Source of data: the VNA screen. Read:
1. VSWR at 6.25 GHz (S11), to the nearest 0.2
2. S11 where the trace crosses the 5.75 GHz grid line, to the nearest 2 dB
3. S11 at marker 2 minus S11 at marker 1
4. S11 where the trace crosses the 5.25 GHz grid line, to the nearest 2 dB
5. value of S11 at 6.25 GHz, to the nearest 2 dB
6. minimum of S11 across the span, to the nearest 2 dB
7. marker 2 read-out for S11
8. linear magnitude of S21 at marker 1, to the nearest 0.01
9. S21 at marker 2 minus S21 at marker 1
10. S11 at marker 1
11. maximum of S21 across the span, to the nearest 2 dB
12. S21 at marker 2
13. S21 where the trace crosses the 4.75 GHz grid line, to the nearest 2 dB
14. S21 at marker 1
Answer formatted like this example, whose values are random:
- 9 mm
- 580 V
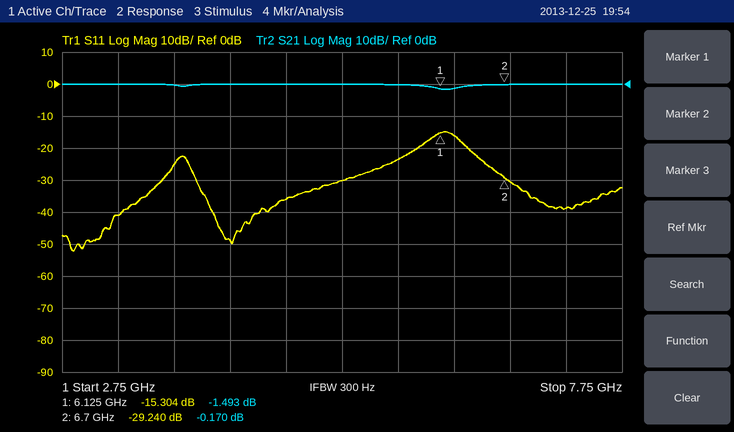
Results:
- 1.4
- -24 dB
- -13.936 dB
- -30 dB
- -16 dB
- -52 dB
- -29.240 dB
- 0.84
- 1.323 dB
- -15.304 dB
- 0 dB
- -0.170 dB
- 0 dB
- -1.493 dB
